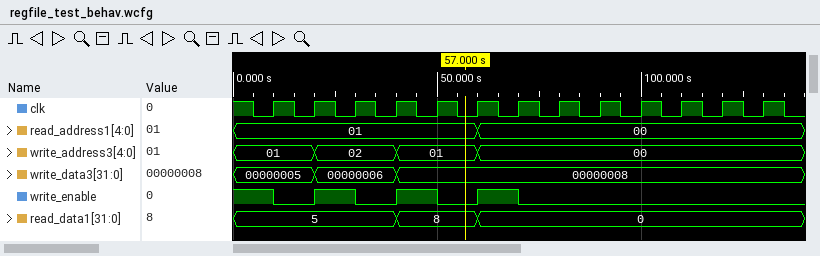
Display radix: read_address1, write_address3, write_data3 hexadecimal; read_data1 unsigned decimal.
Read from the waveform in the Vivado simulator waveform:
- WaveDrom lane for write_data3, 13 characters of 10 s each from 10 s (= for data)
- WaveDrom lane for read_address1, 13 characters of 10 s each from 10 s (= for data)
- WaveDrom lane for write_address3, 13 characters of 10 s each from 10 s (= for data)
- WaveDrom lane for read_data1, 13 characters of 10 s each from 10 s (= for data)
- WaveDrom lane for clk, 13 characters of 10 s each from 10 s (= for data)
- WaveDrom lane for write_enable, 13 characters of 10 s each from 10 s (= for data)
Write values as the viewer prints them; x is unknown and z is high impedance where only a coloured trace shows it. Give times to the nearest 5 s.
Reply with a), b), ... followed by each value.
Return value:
a) {name: 'write_data3', wave: '==.=.........', data: '00000005 00000006 00000008'}
b) {name: 'read_address1', wave: '=....=.......', data: '01 00'}
c) {name: 'write_address3', wave: '==.=.=.......', data: '01 02 01 00'}
d) {name: 'read_data1', wave: '=..=.=.......', data: '5 8 0'}
e) {name: 'clk', wave: 'p............'}
f) {name: 'write_enable', wave: '0101010......'}
